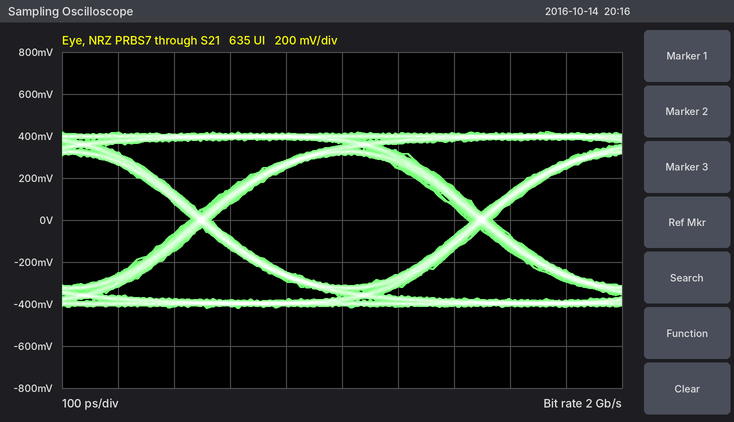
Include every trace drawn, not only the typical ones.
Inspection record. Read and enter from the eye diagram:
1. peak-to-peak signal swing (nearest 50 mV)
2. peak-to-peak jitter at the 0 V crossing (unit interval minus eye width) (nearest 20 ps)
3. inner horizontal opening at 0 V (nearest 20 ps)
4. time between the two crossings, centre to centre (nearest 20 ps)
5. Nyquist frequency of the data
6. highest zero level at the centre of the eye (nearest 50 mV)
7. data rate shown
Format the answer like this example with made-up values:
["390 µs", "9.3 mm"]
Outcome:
["850 mV", "40 ps", "460 ps", "500 ps", "1 GHz", "-300 mV", "2 Gb/s"]
